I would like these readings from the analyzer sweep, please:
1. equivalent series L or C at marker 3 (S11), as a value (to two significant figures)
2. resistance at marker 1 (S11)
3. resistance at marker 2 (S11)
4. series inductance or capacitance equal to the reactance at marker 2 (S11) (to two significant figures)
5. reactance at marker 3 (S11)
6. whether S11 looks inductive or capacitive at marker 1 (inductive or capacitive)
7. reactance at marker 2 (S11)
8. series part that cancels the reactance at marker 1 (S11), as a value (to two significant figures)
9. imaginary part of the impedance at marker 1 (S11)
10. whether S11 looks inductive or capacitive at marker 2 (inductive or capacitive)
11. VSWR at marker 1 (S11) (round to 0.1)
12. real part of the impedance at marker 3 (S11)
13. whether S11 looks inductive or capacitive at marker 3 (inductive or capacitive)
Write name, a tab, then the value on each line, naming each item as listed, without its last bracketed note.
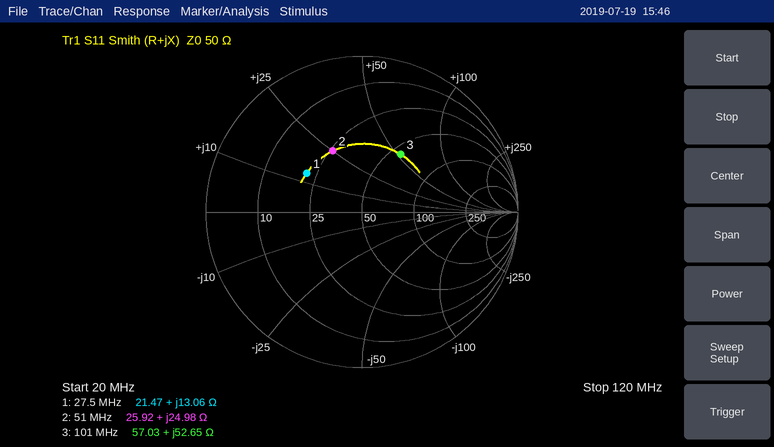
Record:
equivalent series L or C at marker 3 (S11), as a value	83 nH
resistance at marker 1	21.47 Ω
resistance at marker 2	25.92 Ω
series inductance or capacitance equal to the reactance at marker 2 (S11)	78 nH
reactance at marker 3	+52.65 Ω
whether S11 looks inductive or capacitive at marker 1	inductive
reactance at marker 2	+24.98 Ω
series part that cancels the reactance at marker 1 (S11), as a value	440 pF
imaginary part of the impedance at marker 1	+13.06 Ω
whether S11 looks inductive or capacitive at marker 2	inductive
VSWR at marker 1 (S11)	2.5
real part of the impedance at marker 3	57.03 Ω
whether S11 looks inductive or capacitive at marker 3	inductive
